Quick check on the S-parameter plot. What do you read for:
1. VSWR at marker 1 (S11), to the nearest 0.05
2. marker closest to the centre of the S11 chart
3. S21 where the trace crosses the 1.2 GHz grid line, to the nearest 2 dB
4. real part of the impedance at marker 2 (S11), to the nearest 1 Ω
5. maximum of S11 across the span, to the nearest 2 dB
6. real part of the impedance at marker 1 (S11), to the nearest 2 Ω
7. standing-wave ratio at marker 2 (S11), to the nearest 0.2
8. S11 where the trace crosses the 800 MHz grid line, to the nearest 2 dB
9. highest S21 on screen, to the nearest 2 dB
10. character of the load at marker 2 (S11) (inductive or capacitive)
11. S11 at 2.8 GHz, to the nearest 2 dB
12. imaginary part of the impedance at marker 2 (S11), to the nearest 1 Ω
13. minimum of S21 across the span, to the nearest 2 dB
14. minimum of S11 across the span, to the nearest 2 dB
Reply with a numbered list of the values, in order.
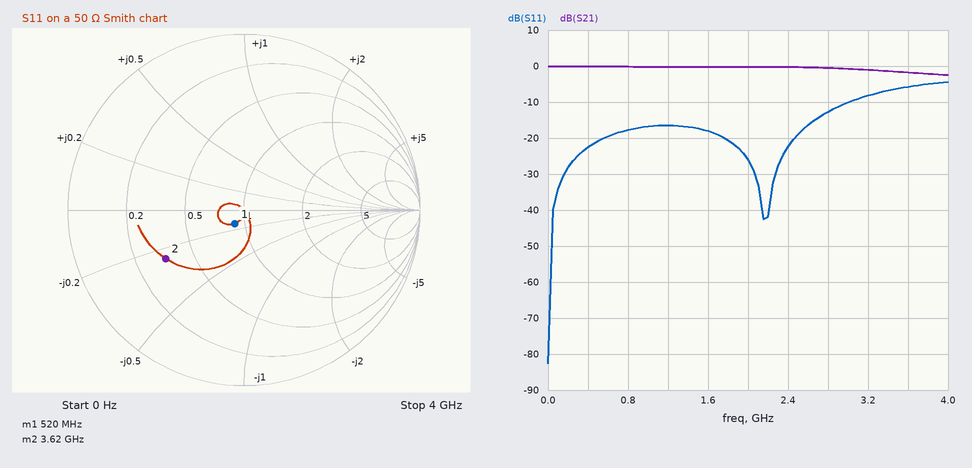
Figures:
1. 1.20
2. marker 1
3. 0 dB
4. 17 Ω
5. -4 dB
6. 44 Ω
7. 3.2
8. -18 dB
9. 0 dB
10. capacitive
11. -12 dB
12. -13 Ω
13. -2 dB
14. -82 dB
